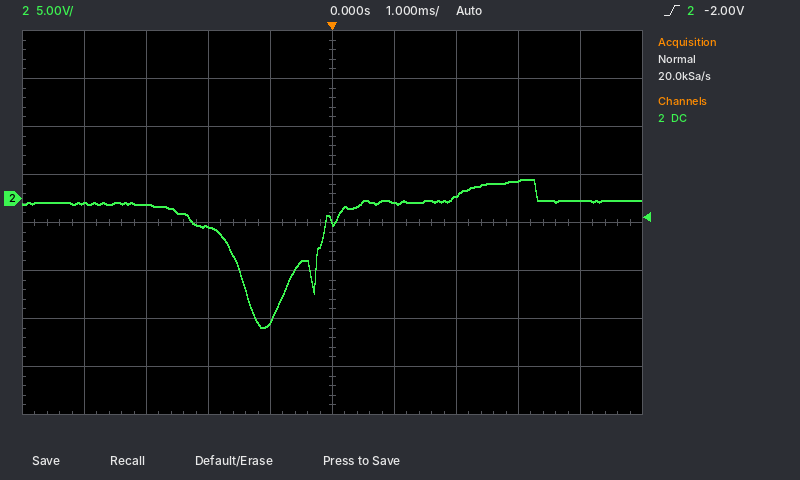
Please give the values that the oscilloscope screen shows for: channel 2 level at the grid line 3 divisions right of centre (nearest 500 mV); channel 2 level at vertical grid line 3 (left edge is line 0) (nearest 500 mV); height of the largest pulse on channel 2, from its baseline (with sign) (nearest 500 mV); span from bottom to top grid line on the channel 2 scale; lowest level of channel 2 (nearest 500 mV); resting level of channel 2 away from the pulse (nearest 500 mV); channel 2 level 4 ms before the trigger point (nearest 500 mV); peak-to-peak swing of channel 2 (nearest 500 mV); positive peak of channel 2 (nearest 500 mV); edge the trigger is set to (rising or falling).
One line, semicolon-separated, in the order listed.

2.0 V; -3.0 V; -13.0 V; 40 V; -13.5 V; -500 mV; -500 mV; 15.5 V; 2.0 V; rising
